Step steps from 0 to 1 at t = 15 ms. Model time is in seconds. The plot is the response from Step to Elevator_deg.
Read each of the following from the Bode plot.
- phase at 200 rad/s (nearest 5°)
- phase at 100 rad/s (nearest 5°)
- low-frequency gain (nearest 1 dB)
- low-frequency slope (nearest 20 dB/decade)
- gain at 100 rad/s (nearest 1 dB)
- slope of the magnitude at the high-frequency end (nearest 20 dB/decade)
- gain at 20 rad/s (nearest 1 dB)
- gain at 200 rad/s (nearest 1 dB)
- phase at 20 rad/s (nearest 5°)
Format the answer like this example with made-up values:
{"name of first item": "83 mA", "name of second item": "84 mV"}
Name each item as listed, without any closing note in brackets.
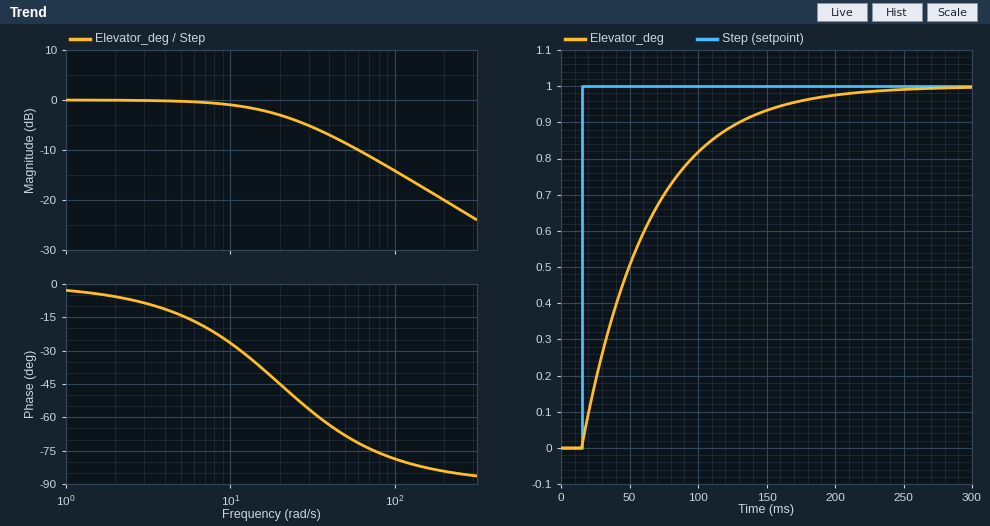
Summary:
{"phase at 200 rad/s": "-85°", "phase at 100 rad/s": "-80°", "low-frequency gain": "0 dB", "low-frequency slope": "0 dB/decade", "gain at 100 rad/s": "-14 dB", "slope of the magnitude at the high-frequency end": "-20 dB/decade", "gain at 20 rad/s": "-3 dB", "gain at 200 rad/s": "-20 dB", "phase at 20 rad/s": "-45°"}
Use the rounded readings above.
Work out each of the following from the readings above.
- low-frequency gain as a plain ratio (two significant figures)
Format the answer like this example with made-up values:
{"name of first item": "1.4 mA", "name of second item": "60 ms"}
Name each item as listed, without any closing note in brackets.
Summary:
{"low-frequency gain as a plain ratio": "1.0"}
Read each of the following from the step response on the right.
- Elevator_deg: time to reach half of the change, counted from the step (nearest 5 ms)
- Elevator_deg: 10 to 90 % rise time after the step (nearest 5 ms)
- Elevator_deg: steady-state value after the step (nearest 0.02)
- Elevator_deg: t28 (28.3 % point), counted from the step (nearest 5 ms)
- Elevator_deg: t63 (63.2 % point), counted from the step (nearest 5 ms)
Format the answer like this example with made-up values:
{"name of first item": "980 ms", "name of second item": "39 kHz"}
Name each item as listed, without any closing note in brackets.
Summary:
{"Elevator_deg: time to reach half of the change, counted from the step": "35 ms", "Elevator_deg: 10 to 90 % rise time after the step": "110 ms", "Elevator_deg: steady-state value after the step": "1.00", "Elevator_deg: t28 (28.3 % point), counted from the step": "15 ms", "Elevator_deg: t63 (63.2 % point), counted from the step": "50 ms"}
